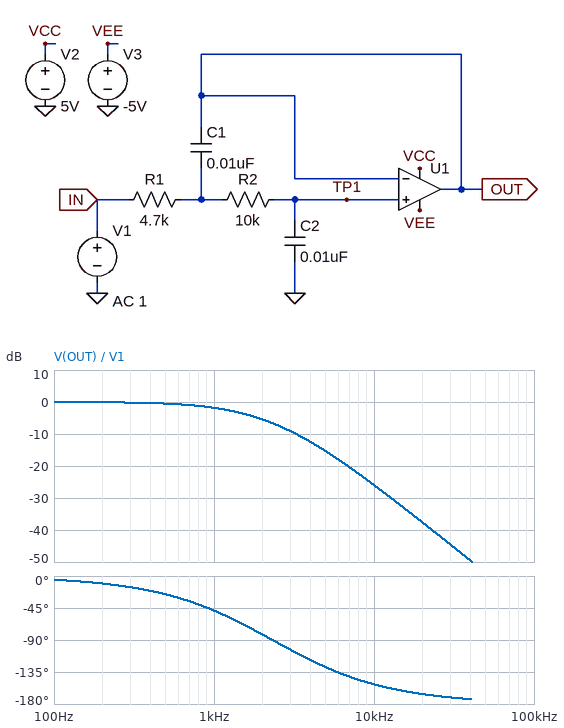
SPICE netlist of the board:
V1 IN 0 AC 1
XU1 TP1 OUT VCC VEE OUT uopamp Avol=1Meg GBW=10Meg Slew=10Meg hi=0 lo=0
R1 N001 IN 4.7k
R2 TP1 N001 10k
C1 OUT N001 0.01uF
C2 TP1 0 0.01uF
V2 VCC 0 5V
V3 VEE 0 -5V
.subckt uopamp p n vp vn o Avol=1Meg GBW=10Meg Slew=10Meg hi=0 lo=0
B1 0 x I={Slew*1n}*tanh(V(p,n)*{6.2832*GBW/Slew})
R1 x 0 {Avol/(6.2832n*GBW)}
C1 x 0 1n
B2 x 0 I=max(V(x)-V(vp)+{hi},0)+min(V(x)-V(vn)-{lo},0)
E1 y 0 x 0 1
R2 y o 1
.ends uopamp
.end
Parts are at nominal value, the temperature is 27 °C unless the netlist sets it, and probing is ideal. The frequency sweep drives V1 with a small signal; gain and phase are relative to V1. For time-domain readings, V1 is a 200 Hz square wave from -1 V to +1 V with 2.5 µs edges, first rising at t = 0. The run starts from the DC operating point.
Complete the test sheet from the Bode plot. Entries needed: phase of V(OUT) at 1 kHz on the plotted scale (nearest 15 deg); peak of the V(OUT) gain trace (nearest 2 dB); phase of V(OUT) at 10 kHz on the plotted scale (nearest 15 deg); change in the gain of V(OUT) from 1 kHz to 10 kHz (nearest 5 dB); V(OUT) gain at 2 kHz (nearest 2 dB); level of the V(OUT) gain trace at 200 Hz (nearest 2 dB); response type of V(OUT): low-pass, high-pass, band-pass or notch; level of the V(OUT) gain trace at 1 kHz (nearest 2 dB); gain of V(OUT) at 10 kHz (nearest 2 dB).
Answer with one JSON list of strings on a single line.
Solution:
["-45 deg", "0 dB", "-150 deg", "-25 dB", "-6 dB", "0 dB", "low-pass", "-2 dB", "-26 dB"]
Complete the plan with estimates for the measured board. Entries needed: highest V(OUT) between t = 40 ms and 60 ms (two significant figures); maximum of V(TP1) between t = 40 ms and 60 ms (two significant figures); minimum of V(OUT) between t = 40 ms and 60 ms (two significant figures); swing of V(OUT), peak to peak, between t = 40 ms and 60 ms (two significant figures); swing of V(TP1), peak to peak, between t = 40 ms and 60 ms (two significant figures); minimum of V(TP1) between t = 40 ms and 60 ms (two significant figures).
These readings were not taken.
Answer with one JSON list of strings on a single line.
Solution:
["1.0 V", "1.0 V", "-1.0 V", "2.0 V", "2.0 V", "-1.0 V"]
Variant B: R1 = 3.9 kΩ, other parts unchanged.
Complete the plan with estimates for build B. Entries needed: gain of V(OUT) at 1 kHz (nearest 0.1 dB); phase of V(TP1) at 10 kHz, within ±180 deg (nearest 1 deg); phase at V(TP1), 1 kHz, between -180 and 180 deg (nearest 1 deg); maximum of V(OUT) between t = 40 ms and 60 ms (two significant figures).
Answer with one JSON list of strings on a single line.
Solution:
["-1.7 dB", "-149 deg", "-46 deg", "1.0 V"]
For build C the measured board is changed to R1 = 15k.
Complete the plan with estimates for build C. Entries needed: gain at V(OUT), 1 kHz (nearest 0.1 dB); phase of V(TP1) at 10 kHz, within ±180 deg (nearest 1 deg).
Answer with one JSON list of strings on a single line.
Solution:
["-4.2 dB", "-165 deg"]
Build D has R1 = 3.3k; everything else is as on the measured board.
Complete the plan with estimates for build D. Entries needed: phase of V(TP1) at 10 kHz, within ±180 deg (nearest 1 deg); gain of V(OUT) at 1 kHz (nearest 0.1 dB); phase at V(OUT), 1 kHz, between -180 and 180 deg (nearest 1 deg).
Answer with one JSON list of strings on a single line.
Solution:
["-145 deg", "-1.6 dB", "-44 deg"]
